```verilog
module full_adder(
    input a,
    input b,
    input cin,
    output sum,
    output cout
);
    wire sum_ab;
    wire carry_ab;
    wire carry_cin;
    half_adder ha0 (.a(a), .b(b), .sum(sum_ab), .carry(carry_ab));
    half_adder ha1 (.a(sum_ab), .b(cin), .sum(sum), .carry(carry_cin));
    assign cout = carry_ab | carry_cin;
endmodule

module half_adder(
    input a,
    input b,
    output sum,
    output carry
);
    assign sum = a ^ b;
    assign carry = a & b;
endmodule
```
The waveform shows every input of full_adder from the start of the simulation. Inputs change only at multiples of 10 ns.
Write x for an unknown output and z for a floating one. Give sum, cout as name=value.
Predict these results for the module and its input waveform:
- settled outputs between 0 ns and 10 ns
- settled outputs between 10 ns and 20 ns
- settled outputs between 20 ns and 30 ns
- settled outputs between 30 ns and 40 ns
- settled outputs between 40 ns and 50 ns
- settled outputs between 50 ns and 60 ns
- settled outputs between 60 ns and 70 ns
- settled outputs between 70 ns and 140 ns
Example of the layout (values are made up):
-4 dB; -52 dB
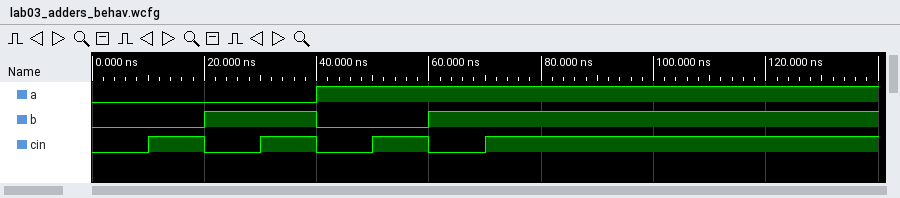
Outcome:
sum=0, cout=0; sum=1, cout=0; sum=1, cout=0; sum=0, cout=1; sum=1, cout=0; sum=0, cout=1; sum=0, cout=1; sum=1, cout=1
